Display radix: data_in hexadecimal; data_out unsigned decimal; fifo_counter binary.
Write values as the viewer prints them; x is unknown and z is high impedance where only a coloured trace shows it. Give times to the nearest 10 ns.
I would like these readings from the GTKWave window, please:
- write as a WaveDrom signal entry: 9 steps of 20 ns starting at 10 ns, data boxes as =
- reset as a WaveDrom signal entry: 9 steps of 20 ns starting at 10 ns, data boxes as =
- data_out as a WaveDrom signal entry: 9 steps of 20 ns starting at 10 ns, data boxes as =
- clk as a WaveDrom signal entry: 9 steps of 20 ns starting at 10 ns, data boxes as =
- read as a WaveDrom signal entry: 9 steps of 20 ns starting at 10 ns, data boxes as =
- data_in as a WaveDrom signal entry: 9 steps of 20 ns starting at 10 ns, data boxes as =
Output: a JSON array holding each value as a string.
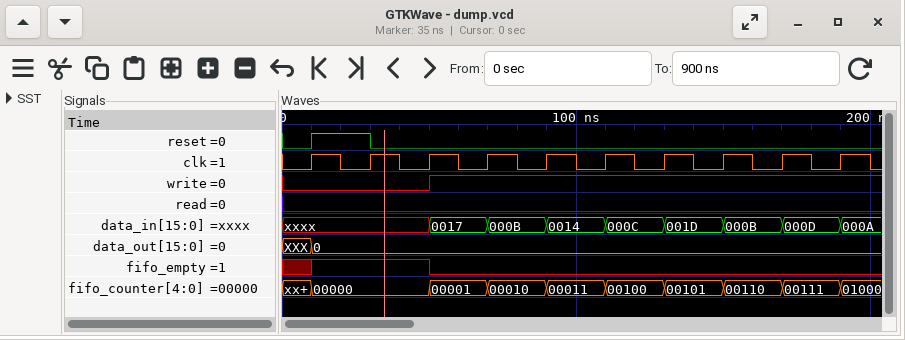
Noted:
["{name: 'write', wave: '0.1......'}", "{name: 'reset', wave: '10.......'}", "{name: 'data_out', wave: '=........', data: '0'}", "{name: 'clk', wave: 'p........'}", "{name: 'read', wave: '0........'}", "{name: 'data_in', wave: 'x.=======', data: '0017 000B 0014 000C 001D 000B 000D'}"]
